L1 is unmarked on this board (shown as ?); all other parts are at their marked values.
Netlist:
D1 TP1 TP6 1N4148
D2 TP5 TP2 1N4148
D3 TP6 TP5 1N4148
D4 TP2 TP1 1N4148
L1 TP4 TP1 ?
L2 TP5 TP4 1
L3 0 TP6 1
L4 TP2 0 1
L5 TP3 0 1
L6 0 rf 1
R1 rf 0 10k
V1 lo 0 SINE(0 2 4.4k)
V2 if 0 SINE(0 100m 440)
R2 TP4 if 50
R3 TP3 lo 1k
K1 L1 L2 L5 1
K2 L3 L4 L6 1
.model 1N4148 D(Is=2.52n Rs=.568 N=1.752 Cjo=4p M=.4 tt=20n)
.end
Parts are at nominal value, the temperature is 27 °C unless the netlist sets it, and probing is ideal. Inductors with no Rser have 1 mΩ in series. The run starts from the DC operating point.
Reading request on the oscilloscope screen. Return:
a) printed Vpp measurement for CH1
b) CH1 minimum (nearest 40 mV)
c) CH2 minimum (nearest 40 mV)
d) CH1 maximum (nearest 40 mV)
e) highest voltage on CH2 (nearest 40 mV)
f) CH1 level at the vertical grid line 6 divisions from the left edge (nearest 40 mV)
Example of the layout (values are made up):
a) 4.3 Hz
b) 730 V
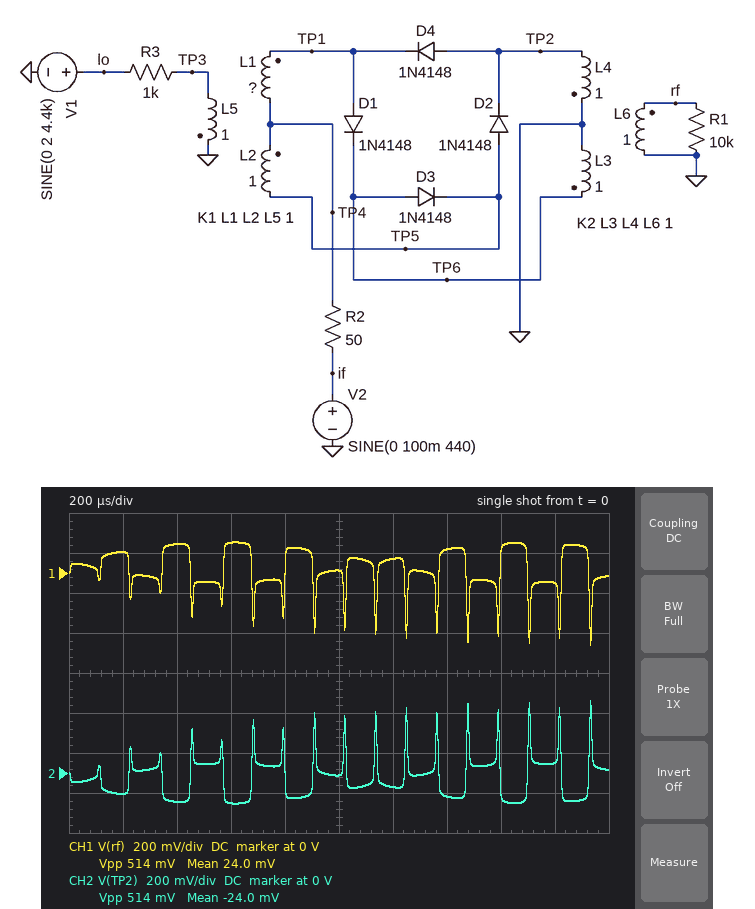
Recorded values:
a) 514 mV
b) -360 mV
c) -160 mV
d) 160 mV
e) 360 mV
f) 80 mV
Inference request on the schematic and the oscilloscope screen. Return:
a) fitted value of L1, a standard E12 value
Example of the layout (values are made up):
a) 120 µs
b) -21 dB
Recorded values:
a) 1.5 H
